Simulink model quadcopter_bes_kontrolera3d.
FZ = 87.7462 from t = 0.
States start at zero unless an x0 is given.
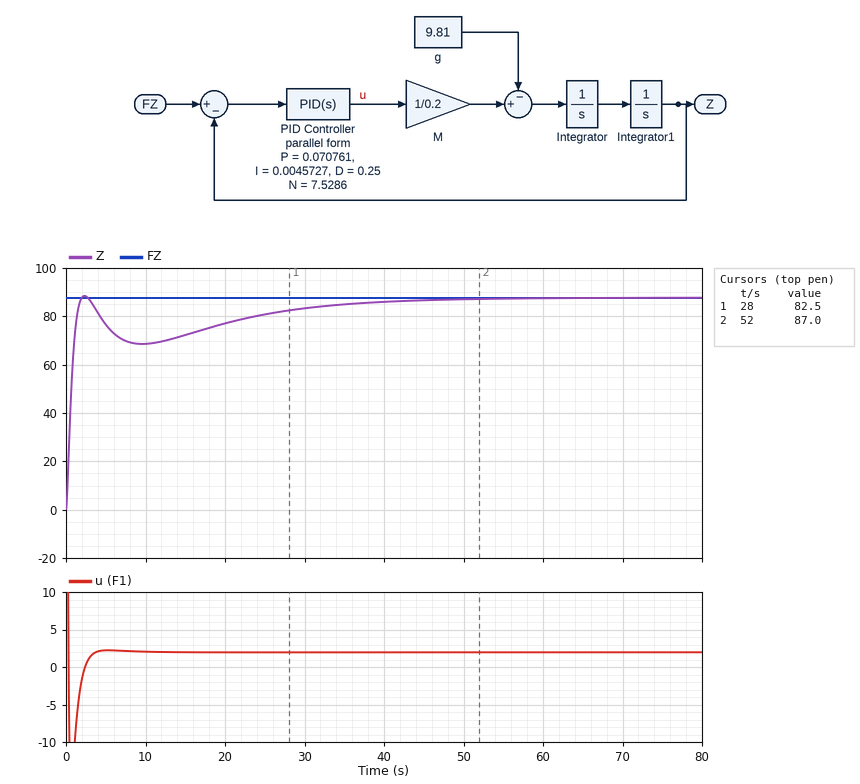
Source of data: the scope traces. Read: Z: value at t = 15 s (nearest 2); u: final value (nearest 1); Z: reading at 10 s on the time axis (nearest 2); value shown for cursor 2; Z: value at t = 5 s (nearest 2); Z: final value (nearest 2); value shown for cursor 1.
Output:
72
2
68
87.0
76
88
82.5
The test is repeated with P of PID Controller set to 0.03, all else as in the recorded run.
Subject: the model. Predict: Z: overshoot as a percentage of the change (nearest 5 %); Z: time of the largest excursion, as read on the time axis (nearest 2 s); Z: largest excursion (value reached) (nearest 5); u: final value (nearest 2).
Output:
10 %
36 s
95
2
